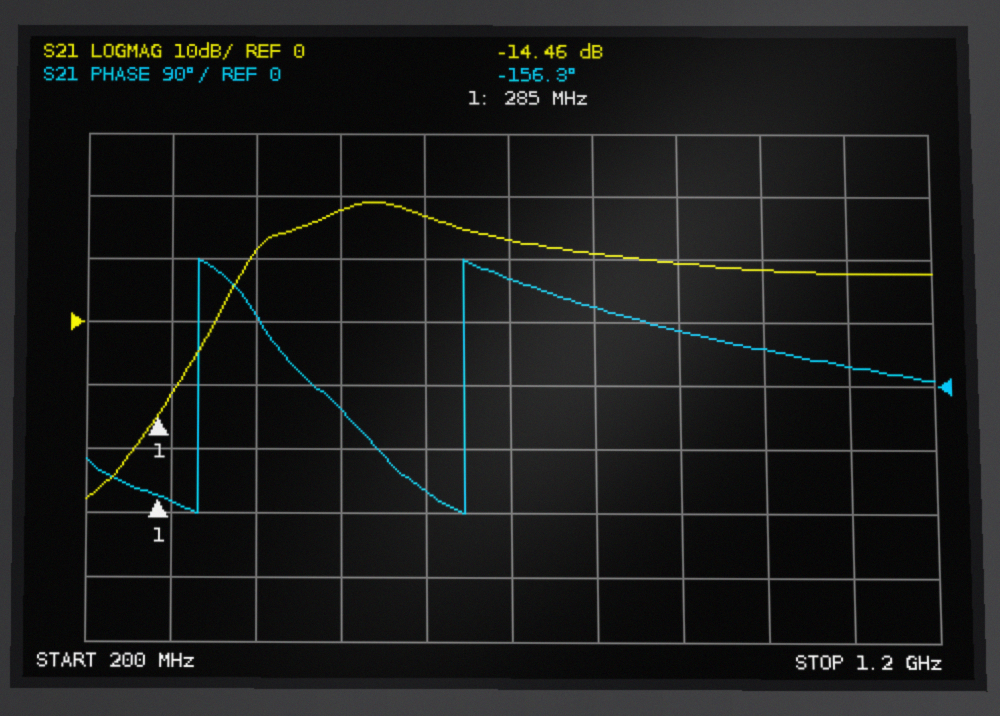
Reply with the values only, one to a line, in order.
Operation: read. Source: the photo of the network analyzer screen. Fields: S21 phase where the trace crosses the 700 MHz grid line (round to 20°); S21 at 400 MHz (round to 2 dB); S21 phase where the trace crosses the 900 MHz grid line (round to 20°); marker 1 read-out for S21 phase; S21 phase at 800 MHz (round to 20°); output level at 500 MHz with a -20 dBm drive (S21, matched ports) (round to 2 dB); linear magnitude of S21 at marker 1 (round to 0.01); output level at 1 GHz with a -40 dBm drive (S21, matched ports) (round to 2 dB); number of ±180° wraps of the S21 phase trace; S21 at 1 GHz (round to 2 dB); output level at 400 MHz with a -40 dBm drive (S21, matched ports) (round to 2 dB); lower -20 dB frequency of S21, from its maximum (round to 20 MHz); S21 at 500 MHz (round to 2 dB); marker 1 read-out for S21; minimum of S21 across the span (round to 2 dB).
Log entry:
160°
12 dB
80°
-156.3°
120°
-2 dBm
0.19
-32 dBm
2
8 dB
-28 dBm
340 MHz
18 dB
-14.46 dB
-28 dB
